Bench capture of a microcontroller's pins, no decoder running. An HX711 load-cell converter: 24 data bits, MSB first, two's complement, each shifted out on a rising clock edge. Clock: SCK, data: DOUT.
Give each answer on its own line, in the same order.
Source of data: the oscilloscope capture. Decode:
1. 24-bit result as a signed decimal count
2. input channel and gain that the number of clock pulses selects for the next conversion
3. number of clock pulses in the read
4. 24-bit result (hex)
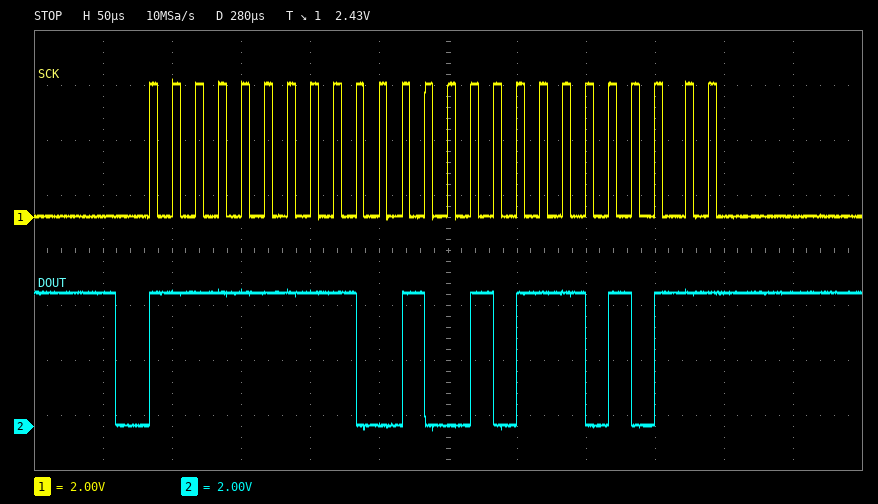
-27925
channel A, gain 128
25
0xFF92EB
